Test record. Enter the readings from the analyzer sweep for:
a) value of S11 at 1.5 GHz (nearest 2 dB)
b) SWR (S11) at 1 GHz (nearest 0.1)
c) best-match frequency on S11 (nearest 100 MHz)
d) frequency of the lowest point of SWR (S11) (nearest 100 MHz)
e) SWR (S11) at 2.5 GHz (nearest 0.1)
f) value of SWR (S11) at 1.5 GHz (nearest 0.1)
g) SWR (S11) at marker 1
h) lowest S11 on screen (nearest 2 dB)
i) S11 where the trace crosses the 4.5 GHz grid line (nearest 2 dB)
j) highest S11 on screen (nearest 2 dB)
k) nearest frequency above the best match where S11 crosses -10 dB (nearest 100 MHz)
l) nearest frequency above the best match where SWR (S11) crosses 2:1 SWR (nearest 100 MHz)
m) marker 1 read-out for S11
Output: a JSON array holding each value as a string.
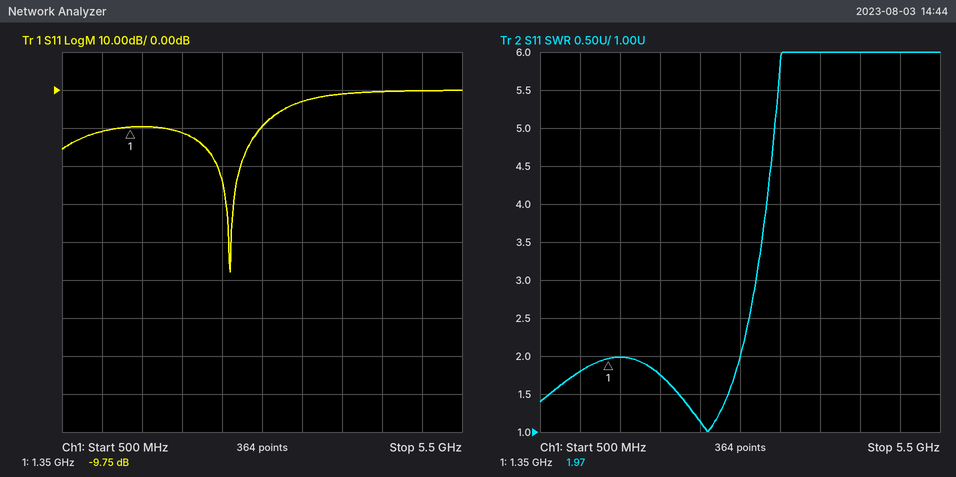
["-10 dB", "1.8", "2.6 GHz", "2.6 GHz", "1.1", "2.0", "1.97", "-48 dB", "0 dB", "0 dB", "3.0 GHz", "3.0 GHz", "-9.75 dB"]
